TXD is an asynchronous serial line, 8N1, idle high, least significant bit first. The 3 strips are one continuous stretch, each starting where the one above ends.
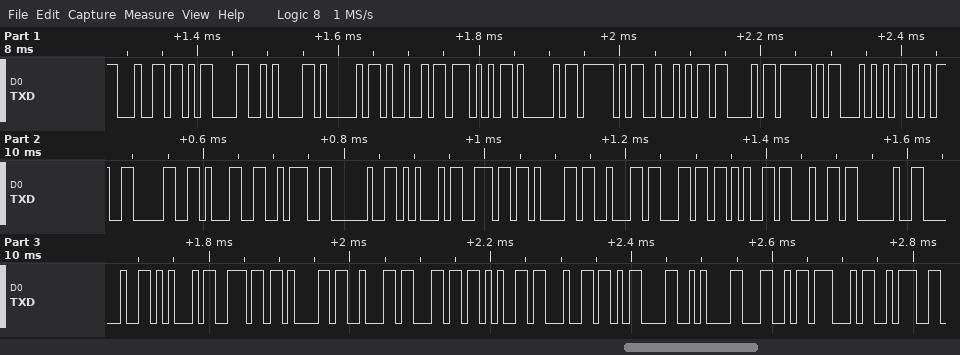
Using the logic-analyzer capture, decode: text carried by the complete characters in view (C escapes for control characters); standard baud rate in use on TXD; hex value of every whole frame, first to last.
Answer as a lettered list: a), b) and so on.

a) "d\r\nAIWA_RC_T501: Enabled  Enabled\r\nLG:"
b) 115200 baud
c) 0x64 0x0D 0x0A 0x41 0x49 0x57 0x41 0x5F 0x52 0x43 0x5F 0x54 0x35 0x30 0x31 0x3A 0x20 0x45 0x6E 0x61 0x62 0x6C 0x65 0x64 0x20 0x20 0x45 0x6E 0x61 0x62 0x6C 0x65 0x64 0x0D 0x0A 0x4C 0x47 0x3A
